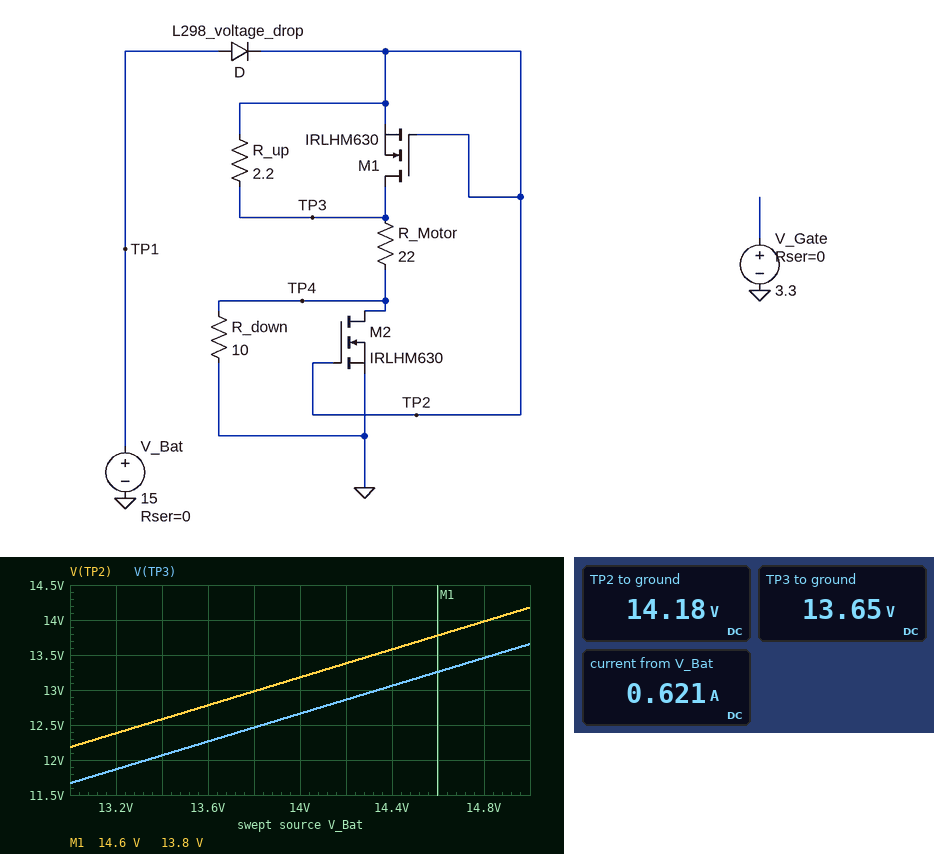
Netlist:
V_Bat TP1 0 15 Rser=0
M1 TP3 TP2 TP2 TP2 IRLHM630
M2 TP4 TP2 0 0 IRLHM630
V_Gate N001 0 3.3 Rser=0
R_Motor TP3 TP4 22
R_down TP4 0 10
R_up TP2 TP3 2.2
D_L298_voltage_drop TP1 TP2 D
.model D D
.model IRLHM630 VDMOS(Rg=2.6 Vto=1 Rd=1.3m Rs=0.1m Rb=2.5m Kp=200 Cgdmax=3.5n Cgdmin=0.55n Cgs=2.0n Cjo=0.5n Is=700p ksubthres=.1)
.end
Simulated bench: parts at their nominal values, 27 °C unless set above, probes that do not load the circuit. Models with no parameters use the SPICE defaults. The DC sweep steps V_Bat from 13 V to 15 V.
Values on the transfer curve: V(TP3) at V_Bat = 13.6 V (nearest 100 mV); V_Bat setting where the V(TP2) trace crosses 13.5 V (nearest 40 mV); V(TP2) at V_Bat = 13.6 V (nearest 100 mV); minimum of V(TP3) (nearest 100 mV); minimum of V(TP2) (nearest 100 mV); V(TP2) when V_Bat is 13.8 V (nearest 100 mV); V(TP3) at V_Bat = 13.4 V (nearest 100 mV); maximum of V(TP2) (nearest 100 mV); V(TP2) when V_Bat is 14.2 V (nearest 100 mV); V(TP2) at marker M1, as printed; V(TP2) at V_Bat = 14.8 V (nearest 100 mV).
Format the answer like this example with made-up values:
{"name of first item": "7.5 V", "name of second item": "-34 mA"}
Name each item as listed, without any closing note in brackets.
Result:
{"V(TP3) at V_Bat = 13.6 V": "12.3 V", "V_Bat setting where the V(TP2) trace crosses 13.5 V": "14.32 V", "V(TP2) at V_Bat = 13.6 V": "12.8 V", "minimum of V(TP3)": "11.7 V", "minimum of V(TP2)": "12.2 V", "V(TP2) when V_Bat is 13.8 V": "13.0 V", "V(TP3) at V_Bat = 13.4 V": "12.1 V", "maximum of V(TP2)": "14.2 V", "V(TP2) when V_Bat is 14.2 V": "13.4 V", "V(TP2) at marker M1, as printed": "13.8 V", "V(TP2) at V_Bat = 14.8 V": "14.0 V"}
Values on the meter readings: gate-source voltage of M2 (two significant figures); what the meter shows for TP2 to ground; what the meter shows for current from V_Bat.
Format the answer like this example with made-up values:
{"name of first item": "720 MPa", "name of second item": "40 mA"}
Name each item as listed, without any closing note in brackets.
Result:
{"gate-source voltage of M2": "14 V", "what the meter shows for TP2 to ground": "14.18 V", "what the meter shows for current from V_Bat": "0.621 A"}
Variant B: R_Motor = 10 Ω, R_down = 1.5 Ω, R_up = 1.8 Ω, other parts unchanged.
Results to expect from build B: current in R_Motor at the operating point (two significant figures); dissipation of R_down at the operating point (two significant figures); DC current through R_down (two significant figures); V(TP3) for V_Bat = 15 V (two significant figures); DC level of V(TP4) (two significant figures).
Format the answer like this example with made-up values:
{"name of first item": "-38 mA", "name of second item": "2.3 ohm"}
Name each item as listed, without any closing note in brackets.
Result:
{"current in R_Motor at the operating point": "1.4 A", "dissipation of R_down at the operating point": "3.9 µW", "DC current through R_down": "1.6 mA", "V(TP3) for V_Bat = 15 V": "14 V", "DC level of V(TP4)": "2.4 mV"}
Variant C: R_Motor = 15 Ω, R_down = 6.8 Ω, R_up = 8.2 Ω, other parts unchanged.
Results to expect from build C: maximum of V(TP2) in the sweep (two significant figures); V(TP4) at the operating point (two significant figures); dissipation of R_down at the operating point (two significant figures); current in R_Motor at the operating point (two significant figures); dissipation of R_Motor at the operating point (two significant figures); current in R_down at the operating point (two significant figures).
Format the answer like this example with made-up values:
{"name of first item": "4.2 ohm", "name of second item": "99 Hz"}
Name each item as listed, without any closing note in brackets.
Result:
{"maximum of V(TP2) in the sweep": "14 V", "V(TP4) at the operating point": "1.6 mV", "dissipation of R_down at the operating point": "380 nW", "current in R_Motor at the operating point": "910 mA", "dissipation of R_Motor at the operating point": "12 W", "current in R_down at the operating point": "240 µA"}
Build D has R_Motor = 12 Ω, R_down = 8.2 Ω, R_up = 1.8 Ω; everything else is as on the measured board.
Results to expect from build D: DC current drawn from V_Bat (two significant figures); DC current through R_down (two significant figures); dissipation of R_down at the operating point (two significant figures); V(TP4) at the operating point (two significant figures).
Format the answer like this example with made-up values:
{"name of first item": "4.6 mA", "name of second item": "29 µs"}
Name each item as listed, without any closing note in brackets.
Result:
{"DC current drawn from V_Bat": "1.1 A", "DC current through R_down": "250 µA", "dissipation of R_down at the operating point": "500 nW", "V(TP4) at the operating point": "2.0 mV"}
